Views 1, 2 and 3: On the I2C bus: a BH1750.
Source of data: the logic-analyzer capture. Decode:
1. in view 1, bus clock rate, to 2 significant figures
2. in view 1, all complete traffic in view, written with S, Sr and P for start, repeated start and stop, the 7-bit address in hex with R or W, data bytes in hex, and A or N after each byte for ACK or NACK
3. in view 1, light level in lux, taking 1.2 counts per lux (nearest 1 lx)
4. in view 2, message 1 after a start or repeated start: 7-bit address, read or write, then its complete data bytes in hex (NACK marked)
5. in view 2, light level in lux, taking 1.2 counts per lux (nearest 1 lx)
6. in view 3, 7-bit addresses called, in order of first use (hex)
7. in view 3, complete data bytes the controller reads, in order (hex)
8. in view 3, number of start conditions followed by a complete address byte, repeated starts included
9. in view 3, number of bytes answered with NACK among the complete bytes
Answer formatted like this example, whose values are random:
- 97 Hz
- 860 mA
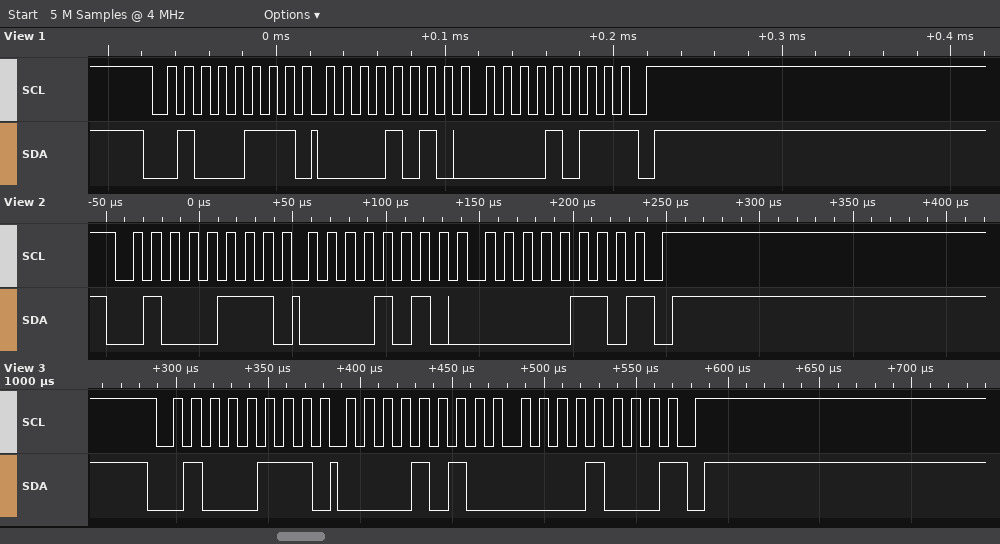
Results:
- 100 kHz
- S 23R A 0A A 0B N P
- 2142 lx
- 0x23 read: 0A 06 NACK
- 2138 lx
- 0x23
- 0A 08
- 1
- 1
